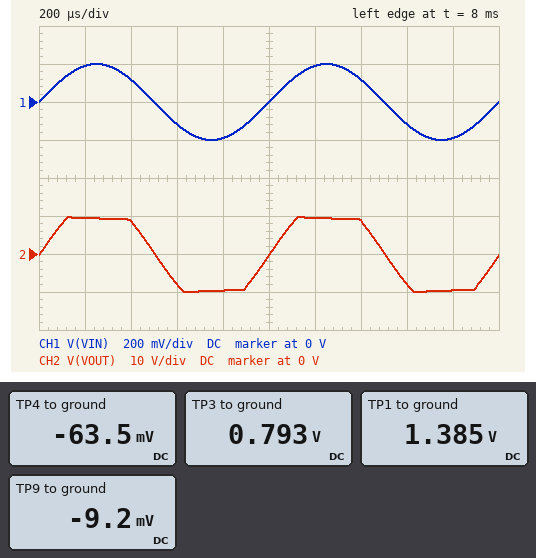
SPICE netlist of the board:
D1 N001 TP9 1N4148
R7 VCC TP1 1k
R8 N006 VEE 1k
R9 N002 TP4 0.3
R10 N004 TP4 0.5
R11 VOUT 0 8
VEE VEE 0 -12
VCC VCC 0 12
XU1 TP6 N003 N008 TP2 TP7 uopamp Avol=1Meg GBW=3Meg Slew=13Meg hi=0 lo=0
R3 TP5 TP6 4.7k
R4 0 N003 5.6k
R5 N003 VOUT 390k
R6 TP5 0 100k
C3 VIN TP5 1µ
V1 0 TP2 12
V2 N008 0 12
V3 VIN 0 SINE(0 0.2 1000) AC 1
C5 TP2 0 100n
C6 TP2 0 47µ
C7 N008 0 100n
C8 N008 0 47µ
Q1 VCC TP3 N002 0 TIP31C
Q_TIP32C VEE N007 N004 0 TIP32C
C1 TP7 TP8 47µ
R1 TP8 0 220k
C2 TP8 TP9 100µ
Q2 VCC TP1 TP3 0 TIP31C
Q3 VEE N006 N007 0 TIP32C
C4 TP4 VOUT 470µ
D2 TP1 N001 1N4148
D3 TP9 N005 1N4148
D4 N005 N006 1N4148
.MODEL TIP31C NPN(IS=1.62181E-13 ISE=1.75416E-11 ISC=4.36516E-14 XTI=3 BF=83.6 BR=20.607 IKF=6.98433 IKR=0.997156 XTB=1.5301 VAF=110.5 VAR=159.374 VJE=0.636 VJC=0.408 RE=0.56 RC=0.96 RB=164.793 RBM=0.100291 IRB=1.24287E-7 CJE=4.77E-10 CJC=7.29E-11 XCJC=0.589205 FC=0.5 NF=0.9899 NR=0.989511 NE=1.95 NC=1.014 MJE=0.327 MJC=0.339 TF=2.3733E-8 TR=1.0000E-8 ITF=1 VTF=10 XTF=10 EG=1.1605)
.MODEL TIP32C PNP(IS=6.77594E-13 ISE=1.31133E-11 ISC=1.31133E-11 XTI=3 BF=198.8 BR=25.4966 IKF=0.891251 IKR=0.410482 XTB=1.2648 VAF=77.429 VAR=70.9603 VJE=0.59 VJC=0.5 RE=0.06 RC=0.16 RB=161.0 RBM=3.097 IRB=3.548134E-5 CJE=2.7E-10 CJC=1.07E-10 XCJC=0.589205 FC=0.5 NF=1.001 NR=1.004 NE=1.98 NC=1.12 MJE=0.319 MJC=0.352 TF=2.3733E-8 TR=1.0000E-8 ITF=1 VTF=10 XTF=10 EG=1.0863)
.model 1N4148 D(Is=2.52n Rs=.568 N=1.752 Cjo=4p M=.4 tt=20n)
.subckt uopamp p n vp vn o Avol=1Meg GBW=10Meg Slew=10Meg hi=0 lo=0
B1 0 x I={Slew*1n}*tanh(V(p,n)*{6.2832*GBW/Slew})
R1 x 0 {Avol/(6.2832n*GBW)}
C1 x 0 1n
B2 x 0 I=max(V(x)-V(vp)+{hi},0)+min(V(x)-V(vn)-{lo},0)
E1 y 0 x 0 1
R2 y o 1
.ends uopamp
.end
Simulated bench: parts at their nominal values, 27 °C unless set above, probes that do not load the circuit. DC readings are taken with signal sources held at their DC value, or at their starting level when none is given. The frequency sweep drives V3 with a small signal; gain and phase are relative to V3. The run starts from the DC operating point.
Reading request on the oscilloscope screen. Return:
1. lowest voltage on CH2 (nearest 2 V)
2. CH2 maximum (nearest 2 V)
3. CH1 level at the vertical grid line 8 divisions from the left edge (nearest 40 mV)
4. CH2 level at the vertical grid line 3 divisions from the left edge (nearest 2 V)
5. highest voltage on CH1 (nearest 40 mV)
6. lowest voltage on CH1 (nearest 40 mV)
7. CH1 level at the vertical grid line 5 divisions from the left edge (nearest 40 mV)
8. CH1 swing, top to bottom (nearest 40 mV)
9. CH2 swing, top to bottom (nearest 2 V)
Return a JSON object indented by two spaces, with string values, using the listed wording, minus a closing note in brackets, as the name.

{
  "lowest voltage on CH2": "-10 V",
  "CH2 maximum": "10 V",
  "CH1 level at the vertical grid line 8 divisions from the left edge": "-120 mV",
  "CH2 level at the vertical grid line 3 divisions from the left edge": "-8 V",
  "highest voltage on CH1": "200 mV",
  "lowest voltage on CH1": "-200 mV",
  "CH1 level at the vertical grid line 5 divisions from the left edge": "0 V",
  "CH1 swing, top to bottom": "400 mV",
  "CH2 swing, top to bottom": "20 V"
}
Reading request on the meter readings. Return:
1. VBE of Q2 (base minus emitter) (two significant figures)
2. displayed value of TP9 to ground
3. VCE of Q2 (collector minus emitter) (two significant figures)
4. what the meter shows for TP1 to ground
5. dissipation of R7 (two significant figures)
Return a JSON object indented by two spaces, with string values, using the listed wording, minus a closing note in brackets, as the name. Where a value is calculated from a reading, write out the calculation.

{
  "VBE of Q2 (base minus emitter)": "1.385 V - 793 mV = 590 mV",
  "displayed value of TP9 to ground": "-9.2 mV",
  "VCE of Q2 (collector minus emitter)": "12 V - 793 mV = 11 V",
  "what the meter shows for TP1 to ground": "1.385 V",
  "dissipation of R7": "(12 V - 1.385 V)^2 / 1 kΩ = 110 mW"
}
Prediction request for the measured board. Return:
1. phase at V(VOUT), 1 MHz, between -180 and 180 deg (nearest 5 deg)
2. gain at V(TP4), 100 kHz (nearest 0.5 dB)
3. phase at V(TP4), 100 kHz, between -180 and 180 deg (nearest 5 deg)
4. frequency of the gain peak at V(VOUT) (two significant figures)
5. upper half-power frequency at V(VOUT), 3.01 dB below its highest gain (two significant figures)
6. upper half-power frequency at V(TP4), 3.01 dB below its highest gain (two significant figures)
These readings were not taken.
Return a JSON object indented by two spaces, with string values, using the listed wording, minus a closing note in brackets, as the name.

{
  "phase at V(VOUT), 1 MHz, between -180 and 180 deg": "-105 deg",
  "gain at V(TP4), 100 kHz": "28.5 dB",
  "phase at V(TP4), 100 kHz, between -180 and 180 deg": "-70 deg",
  "frequency of the gain peak at V(VOUT)": "170 mHz",
  "upper half-power frequency at V(VOUT), 3.01 dB below its highest gain": "180 mHz",
  "upper half-power frequency at V(TP4), 3.01 dB below its highest gain": "180 mHz"
}
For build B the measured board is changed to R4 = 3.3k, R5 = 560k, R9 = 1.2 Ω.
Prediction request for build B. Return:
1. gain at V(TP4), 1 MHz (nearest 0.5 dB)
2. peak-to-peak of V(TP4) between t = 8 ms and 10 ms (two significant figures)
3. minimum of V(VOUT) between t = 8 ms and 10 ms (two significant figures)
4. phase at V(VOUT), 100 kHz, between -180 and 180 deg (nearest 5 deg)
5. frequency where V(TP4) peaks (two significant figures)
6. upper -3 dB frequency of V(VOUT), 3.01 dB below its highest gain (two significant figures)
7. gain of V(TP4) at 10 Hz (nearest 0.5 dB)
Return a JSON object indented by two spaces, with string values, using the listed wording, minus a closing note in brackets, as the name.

{
  "gain at V(TP4), 1 MHz": "7.5 dB",
  "peak-to-peak of V(TP4) between t = 8 ms and 10 ms": "18 V",
  "minimum of V(VOUT) between t = 8 ms and 10 ms": "-9.8 V",
  "phase at V(VOUT), 100 kHz, between -180 and 180 deg": "-85 deg",
  "frequency where V(TP4) peaks": "270 mHz",
  "upper -3 dB frequency of V(VOUT), 3.01 dB below its highest gain": "290 mHz",
  "gain of V(TP4) at 10 Hz": "57.5 dB"
}
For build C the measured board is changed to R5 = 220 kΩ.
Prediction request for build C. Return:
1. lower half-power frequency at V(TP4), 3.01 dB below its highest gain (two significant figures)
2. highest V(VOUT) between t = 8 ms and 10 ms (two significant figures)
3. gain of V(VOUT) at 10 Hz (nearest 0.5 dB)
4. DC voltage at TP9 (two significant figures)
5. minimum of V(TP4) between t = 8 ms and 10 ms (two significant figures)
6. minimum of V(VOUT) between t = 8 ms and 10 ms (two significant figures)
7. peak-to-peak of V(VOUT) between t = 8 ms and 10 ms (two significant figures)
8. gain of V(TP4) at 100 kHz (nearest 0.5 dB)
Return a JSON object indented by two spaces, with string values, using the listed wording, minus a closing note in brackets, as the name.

{
  "lower half-power frequency at V(TP4), 3.01 dB below its highest gain": "130 mHz",
  "highest V(VOUT) between t = 8 ms and 10 ms": "8.0 V",
  "gain of V(VOUT) at 10 Hz": "32.0 dB",
  "DC voltage at TP9": "-9.2 mV",
  "minimum of V(TP4) between t = 8 ms and 10 ms": "-7.8 V",
  "minimum of V(VOUT) between t = 8 ms and 10 ms": "-8.1 V",
  "peak-to-peak of V(VOUT) between t = 8 ms and 10 ms": "16 V",
  "gain of V(TP4) at 100 kHz": "27.5 dB"
}
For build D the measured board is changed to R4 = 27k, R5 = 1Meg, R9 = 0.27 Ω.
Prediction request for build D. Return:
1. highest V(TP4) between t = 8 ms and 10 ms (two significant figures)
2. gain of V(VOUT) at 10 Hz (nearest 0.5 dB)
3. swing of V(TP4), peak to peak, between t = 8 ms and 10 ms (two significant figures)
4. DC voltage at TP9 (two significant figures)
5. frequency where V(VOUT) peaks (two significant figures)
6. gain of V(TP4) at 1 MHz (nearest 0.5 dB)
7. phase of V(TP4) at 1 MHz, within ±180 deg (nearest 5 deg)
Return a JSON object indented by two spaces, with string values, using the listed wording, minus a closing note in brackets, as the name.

{
  "highest V(TP4) between t = 8 ms and 10 ms": "7.8 V",
  "gain of V(VOUT) at 10 Hz": "31.5 dB",
  "swing of V(TP4), peak to peak, between t = 8 ms and 10 ms": "15 V",
  "DC voltage at TP9": "-9.3 mV",
  "frequency where V(VOUT) peaks": "130 mHz",
  "gain of V(TP4) at 1 MHz": "8.5 dB",
  "phase of V(TP4) at 1 MHz, within ±180 deg": "-100 deg"
}
